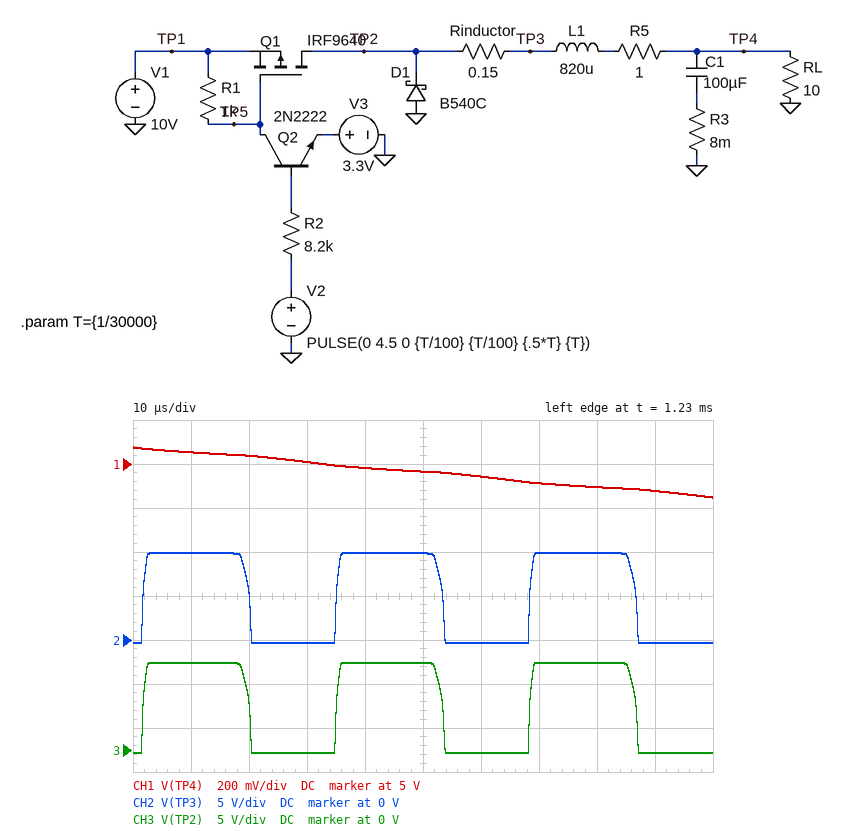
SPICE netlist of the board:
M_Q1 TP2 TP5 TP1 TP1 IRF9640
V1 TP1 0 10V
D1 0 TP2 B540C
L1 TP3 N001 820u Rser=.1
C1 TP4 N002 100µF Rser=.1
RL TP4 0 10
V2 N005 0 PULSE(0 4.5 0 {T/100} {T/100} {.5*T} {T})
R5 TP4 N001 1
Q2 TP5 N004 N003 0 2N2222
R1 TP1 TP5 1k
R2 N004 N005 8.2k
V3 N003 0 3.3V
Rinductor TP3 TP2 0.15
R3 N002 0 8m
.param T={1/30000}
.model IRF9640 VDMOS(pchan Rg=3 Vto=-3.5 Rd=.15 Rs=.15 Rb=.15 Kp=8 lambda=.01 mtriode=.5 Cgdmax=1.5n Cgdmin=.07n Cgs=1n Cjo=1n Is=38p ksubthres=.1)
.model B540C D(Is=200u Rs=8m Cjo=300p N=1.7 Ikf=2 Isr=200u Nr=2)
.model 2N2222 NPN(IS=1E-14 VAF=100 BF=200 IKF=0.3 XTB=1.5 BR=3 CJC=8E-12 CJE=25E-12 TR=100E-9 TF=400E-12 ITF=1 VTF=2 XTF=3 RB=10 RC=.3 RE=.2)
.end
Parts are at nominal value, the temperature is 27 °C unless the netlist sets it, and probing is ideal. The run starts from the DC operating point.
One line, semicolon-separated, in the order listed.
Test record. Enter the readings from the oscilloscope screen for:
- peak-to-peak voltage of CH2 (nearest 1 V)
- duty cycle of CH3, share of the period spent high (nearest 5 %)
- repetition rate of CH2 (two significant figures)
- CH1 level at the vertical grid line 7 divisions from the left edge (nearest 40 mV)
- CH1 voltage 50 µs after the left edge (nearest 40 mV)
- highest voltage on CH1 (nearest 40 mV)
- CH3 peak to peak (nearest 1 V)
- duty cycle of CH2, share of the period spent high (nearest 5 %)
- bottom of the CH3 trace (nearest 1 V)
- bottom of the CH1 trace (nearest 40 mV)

10 V; 55 %; 30 kHz; 4.92 V; 4.96 V; 5.08 V; 10 V; 55 %; 0 V; 4.84 V
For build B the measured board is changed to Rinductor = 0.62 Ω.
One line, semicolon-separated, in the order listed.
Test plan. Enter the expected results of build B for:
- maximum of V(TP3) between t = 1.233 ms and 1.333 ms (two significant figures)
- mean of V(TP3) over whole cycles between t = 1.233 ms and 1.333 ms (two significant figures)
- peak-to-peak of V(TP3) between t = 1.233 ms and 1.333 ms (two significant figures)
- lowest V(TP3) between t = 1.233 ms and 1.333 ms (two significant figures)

9.7 V; 5.0 V; 10 V; -570 mV
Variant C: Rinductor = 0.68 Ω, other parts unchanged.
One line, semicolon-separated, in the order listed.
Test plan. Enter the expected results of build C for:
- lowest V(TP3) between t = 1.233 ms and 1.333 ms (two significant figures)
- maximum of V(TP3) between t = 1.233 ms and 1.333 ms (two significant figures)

-590 mV; 9.7 V
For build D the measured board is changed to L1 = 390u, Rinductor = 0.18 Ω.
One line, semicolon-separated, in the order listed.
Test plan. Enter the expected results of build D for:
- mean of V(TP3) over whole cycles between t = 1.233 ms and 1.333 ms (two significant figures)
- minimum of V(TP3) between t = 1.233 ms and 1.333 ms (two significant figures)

5.0 V; -460 mV
